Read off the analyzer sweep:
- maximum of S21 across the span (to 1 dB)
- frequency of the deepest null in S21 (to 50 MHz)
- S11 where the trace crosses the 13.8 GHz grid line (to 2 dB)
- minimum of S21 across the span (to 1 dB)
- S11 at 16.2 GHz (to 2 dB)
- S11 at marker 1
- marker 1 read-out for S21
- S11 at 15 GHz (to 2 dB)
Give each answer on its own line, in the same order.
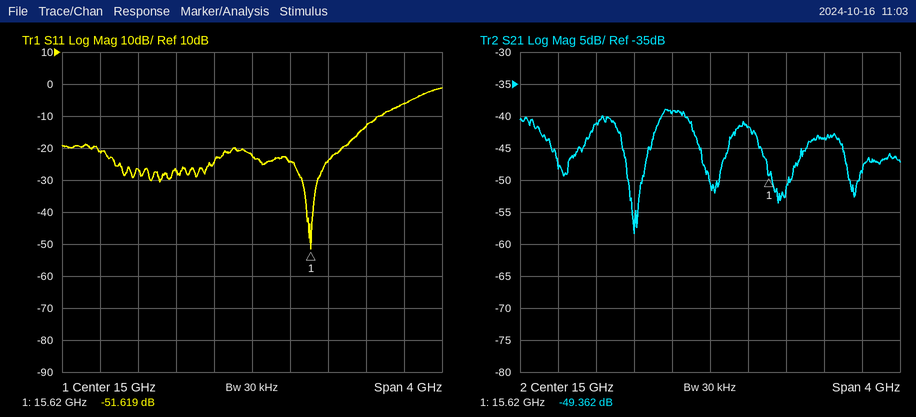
-39 dB
14.20 GHz
-26 dB
-58 dB
-14 dB
-51.619 dB
-49.362 dB
-22 dB
